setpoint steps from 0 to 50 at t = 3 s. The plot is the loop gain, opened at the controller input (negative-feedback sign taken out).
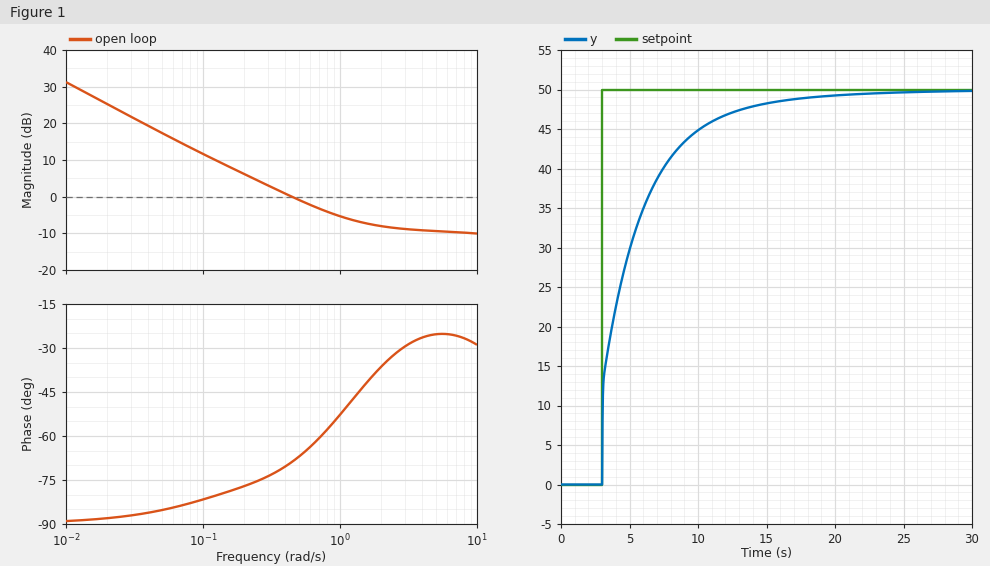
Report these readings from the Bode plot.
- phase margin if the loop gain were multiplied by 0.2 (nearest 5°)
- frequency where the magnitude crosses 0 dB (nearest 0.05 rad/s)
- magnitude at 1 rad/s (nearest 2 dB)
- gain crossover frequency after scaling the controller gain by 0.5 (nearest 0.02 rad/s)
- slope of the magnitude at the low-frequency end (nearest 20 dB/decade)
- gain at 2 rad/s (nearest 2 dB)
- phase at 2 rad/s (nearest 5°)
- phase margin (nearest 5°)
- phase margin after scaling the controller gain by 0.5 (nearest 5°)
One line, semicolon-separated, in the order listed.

95°; 0.45 rad/s; -6 dB; 0.20 rad/s; -20 dB/decade; -8 dB; -35°; 110°; 105°
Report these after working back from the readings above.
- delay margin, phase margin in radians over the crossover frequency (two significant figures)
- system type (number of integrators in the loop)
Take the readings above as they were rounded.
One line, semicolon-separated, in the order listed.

4.3 s; 1
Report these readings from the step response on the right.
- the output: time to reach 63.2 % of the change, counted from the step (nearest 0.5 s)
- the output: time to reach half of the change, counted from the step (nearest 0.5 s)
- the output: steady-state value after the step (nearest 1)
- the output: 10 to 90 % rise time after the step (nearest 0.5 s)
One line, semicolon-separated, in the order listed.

2.5 s; 1.5 s; 50; 7.0 s
